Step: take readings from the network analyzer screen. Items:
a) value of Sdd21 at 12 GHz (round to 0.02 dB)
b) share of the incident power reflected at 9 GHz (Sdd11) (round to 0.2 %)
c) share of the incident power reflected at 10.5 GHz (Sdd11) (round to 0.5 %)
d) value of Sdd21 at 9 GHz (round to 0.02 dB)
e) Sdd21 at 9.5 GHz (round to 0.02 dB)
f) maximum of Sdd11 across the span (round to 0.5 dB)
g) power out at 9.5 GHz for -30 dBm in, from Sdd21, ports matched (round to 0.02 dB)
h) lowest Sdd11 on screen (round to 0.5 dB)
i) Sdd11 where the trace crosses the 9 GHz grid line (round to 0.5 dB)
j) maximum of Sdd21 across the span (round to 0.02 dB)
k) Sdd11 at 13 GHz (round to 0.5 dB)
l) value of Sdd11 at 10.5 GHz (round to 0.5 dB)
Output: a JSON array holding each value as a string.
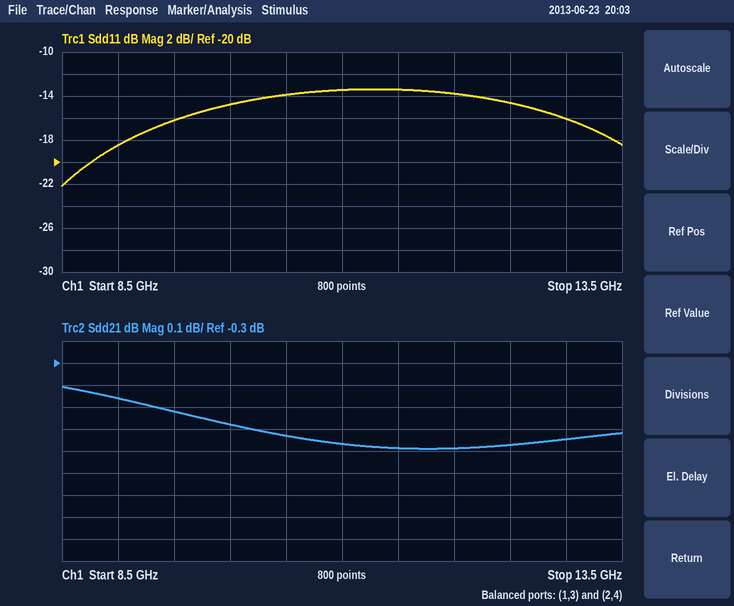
["-0.68 dB", "1.4 %", "4.0 %", "-0.46 dB", "-0.52 dB", "-13.5 dB", "-30.52 dBm", "-22.0 dB", "-18.5 dB", "-0.40 dB", "-16.0 dB", "-14.0 dB"]
